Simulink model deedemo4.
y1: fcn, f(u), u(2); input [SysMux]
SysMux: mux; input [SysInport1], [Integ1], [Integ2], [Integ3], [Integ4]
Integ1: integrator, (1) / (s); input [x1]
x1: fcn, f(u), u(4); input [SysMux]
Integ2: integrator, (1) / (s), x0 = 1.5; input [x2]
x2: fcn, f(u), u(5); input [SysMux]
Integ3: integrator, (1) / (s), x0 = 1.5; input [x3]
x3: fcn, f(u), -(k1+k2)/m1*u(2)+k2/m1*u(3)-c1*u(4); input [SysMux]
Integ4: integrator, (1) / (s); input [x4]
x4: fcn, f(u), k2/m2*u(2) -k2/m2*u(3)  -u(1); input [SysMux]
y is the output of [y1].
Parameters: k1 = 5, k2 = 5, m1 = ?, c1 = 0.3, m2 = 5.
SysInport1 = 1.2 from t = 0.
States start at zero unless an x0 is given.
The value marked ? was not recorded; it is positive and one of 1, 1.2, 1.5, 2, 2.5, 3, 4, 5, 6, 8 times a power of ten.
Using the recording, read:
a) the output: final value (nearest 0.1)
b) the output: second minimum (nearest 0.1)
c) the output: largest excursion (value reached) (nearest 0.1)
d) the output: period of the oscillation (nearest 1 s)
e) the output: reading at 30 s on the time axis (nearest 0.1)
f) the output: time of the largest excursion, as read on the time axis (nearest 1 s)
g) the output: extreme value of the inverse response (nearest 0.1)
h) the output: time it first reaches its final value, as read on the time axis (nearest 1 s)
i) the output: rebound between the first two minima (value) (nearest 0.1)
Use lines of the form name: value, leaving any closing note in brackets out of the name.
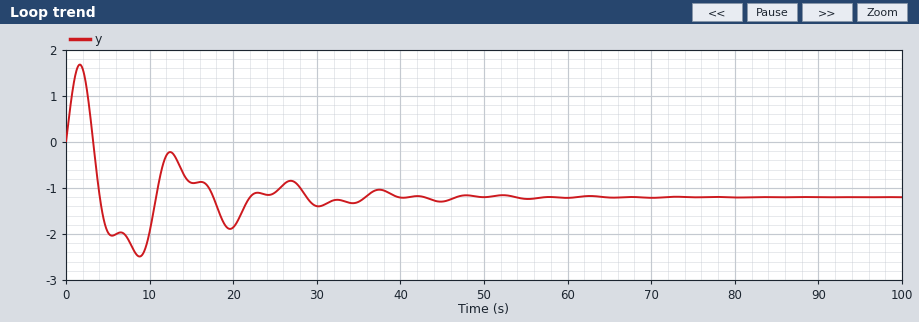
the output: final value: -1.2
the output: second minimum: -1.9
the output: largest excursion (value reached): -2.5
the output: period of the oscillation: 11 s
the output: reading at 30 s on the time axis: -1.4
the output: time of the largest excursion, as read on the time axis: 9 s
the output: extreme value of the inverse response: 1.7
the output: time it first reaches its final value, as read on the time axis: 4 s
the output: rebound between the first two minima (value): -0.2
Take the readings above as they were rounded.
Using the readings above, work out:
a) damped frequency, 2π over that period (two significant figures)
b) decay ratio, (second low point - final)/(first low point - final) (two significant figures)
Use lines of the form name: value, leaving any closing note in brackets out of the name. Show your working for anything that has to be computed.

damped frequency, 2π over that period: 2π / 11 = 0.57 rad/s
decay ratio, (second low point - final)/(first low point - final): (-1.9 - (-1.2)) / (-2.5 - (-1.2)) = 0.54
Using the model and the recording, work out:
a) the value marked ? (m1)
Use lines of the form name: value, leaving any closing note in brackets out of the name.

the value marked ?: 12
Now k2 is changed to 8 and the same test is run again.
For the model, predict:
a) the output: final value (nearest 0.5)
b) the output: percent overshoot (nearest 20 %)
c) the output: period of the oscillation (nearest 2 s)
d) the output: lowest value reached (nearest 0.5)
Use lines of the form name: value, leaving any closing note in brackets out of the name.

the output: final value: -1.0
the output: percent overshoot: 140 %
the output: period of the oscillation: 12 s
the output: lowest value reached: -3.0
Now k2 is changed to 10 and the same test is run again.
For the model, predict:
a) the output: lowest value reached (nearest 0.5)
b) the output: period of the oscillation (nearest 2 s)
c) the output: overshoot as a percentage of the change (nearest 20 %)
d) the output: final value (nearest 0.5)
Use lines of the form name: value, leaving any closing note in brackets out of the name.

the output: lowest value reached: -3.0
the output: period of the oscillation: 8 s
the output: overshoot as a percentage of the change: 140 %
the output: final value: -1.0
